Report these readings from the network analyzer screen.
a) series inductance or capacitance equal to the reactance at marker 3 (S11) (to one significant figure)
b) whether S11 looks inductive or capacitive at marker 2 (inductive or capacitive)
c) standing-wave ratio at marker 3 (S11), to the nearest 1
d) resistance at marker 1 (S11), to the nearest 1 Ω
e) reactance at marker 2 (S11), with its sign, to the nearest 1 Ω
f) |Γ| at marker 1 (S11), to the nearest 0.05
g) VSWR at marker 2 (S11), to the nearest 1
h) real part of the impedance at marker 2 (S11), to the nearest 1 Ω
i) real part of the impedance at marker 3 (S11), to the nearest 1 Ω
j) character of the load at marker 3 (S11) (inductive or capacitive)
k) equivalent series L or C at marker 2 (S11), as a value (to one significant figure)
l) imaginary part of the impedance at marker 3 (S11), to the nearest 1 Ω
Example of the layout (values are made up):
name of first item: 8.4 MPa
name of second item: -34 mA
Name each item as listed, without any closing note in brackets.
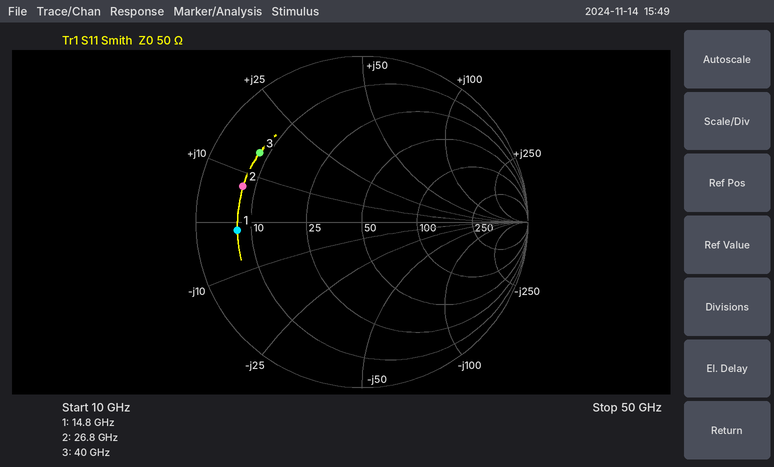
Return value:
series inductance or capacitance equal to the reactance at marker 3 (S11): 60 pH
whether S11 looks inductive or capacitive at marker 2: inductive
standing-wave ratio at marker 3 (S11), to the nearest 1: 7
resistance at marker 1 (S11), to the nearest 1 Ω: 7 Ω
reactance at marker 2 (S11), with its sign, to the nearest 1 Ω: +7 Ω
|Γ| at marker 1 (S11), to the nearest 0.05: 0.75
VSWR at marker 2 (S11), to the nearest 1: 7
real part of the impedance at marker 2 (S11), to the nearest 1 Ω: 7 Ω
real part of the impedance at marker 3 (S11), to the nearest 1 Ω: 8 Ω
character of the load at marker 3 (S11): inductive
equivalent series L or C at marker 2 (S11), as a value: 40 pH
imaginary part of the impedance at marker 3 (S11), to the nearest 1 Ω: +15 Ω
